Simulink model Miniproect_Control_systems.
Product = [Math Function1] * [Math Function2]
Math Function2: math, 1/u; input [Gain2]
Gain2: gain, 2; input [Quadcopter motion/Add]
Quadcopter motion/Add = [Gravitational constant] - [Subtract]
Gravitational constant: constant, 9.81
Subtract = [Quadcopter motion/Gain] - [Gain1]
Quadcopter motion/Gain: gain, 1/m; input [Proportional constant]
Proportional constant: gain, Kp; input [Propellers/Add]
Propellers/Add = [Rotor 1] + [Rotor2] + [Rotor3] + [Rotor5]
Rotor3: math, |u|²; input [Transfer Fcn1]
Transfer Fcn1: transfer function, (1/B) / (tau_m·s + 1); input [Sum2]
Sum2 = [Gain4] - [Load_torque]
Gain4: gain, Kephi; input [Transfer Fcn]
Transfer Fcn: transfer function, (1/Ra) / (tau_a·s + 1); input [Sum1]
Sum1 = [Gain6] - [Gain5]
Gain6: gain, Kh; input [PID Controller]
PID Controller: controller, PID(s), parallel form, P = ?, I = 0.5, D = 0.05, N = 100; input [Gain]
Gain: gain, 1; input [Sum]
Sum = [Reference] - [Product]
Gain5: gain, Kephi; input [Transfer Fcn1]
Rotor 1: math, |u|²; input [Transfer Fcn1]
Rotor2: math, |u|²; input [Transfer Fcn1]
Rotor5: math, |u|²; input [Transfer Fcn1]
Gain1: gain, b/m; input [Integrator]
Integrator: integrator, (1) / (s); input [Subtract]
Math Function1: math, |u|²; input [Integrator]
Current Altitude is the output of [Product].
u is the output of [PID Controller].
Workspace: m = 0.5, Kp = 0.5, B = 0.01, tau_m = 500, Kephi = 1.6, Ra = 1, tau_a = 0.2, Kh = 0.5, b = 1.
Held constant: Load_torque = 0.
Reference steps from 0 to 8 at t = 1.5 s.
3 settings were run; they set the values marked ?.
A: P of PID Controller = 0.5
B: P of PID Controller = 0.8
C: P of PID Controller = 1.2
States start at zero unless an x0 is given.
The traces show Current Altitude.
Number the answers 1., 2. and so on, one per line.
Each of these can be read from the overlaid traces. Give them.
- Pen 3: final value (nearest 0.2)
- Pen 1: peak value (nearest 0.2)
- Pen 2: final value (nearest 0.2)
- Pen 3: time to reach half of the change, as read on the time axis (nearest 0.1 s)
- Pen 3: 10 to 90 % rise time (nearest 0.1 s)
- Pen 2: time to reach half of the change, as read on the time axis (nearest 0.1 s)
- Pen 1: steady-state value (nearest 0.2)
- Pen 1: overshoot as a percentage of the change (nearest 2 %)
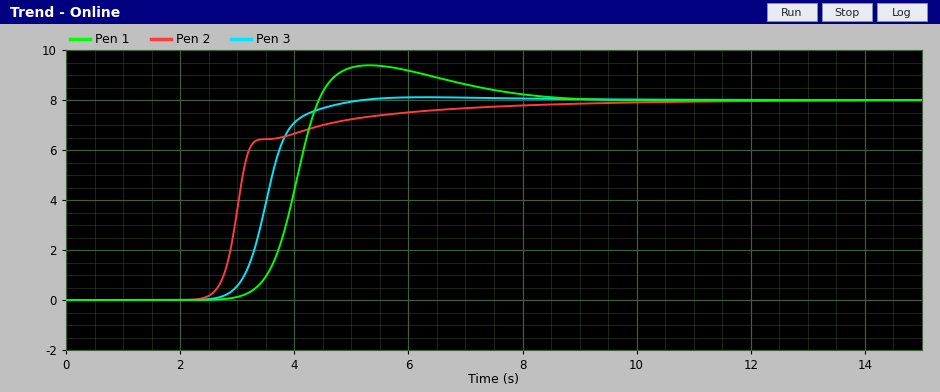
1. 8.0
2. 9.4
3. 8.0
4. 3.5 s
5. 1.0 s
6. 3.0 s
7. 8.0
8. 18 %
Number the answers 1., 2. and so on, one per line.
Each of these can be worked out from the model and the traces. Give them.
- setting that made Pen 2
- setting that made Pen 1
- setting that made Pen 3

1. C
2. A
3. B
